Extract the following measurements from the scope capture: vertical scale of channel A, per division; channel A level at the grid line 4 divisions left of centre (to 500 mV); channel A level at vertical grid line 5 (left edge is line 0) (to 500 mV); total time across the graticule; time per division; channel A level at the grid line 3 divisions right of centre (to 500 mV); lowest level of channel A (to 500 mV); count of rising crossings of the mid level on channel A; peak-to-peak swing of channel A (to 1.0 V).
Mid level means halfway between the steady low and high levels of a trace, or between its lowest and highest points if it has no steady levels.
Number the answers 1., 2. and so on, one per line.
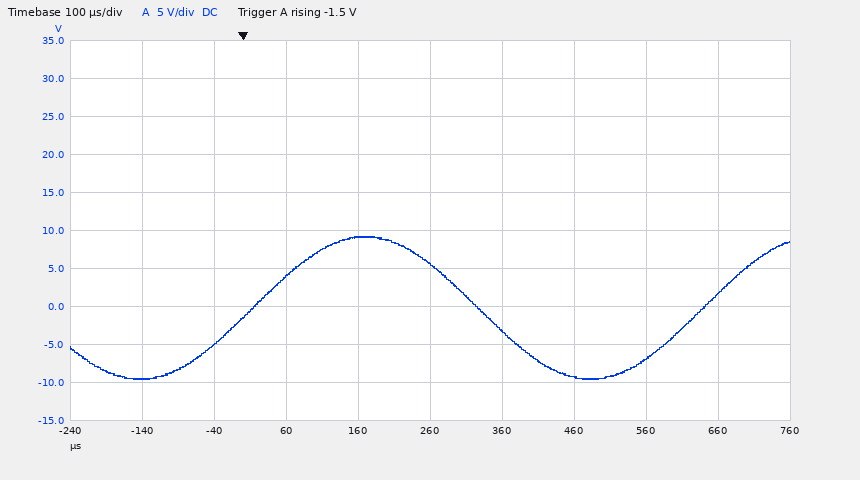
1. 5 V
2. -9.5 V
3. 5.5 V
4. 1 ms
5. 100 µs
6. -7.0 V
7. -9.5 V
8. 2
9. 19.0 V
